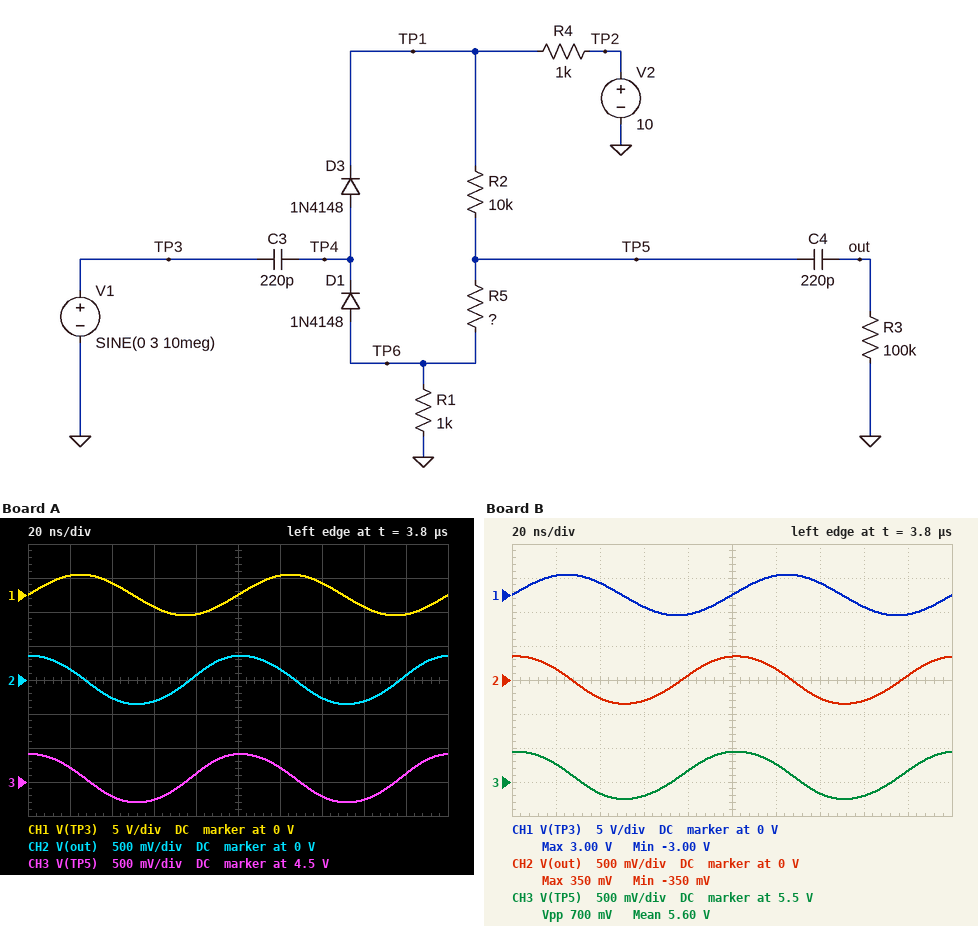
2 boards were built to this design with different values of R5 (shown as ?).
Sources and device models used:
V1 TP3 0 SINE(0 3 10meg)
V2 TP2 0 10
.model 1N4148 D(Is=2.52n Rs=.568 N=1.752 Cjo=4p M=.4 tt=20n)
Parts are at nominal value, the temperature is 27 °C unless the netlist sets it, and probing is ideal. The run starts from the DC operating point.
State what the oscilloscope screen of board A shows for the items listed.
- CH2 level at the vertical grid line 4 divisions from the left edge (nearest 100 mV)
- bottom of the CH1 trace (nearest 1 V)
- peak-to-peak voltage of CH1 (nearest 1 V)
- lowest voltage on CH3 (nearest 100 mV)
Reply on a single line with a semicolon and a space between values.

100 mV; -3 V; 6 V; 4.2 V
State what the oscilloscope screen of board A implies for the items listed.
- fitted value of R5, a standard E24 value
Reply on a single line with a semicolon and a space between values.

8.2 kΩ
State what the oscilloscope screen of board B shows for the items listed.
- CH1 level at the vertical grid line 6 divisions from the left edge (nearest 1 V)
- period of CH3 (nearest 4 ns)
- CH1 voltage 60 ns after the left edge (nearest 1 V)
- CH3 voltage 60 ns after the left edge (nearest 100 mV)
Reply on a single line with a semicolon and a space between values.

3 V; 100 ns; -2 V; 5.3 V
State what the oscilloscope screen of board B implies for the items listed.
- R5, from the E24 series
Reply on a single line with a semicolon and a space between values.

13 kΩ
